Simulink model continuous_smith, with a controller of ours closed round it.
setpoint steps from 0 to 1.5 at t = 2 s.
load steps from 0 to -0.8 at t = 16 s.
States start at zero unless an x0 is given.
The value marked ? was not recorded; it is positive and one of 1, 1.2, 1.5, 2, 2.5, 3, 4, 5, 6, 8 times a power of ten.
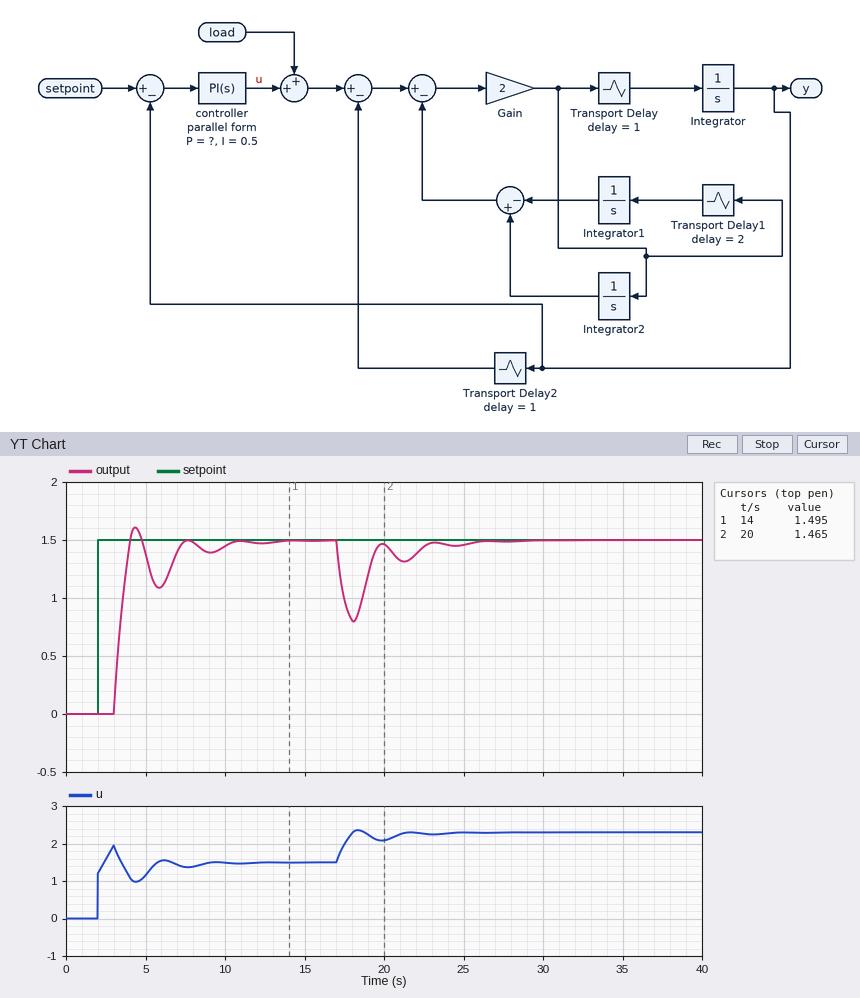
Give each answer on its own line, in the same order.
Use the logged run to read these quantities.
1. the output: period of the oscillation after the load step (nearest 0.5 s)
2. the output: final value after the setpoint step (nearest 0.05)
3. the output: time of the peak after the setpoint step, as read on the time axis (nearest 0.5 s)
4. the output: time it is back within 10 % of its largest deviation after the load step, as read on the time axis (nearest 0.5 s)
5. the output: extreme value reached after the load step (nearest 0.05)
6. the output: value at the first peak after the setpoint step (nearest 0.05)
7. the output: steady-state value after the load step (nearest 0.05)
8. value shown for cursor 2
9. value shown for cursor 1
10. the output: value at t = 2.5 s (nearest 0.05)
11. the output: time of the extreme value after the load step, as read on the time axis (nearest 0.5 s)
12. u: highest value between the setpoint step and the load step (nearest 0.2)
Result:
3.0 s
1.50
4.5 s
22.5 s
0.80
1.60
1.50
1.465
1.495
0.00
18.0 s
2.0
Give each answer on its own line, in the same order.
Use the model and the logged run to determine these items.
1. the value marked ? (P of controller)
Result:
0.8
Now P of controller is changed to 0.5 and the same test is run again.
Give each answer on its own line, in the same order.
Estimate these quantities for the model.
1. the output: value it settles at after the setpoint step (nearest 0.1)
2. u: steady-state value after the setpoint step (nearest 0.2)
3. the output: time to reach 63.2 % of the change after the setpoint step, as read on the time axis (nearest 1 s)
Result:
1.5
1.4
4 s
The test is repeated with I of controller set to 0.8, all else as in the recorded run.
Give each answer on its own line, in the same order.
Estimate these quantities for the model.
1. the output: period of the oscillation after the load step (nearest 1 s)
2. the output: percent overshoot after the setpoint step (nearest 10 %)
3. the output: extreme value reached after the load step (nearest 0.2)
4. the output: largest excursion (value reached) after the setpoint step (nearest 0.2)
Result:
4 s
30 %
0.8
2.0
